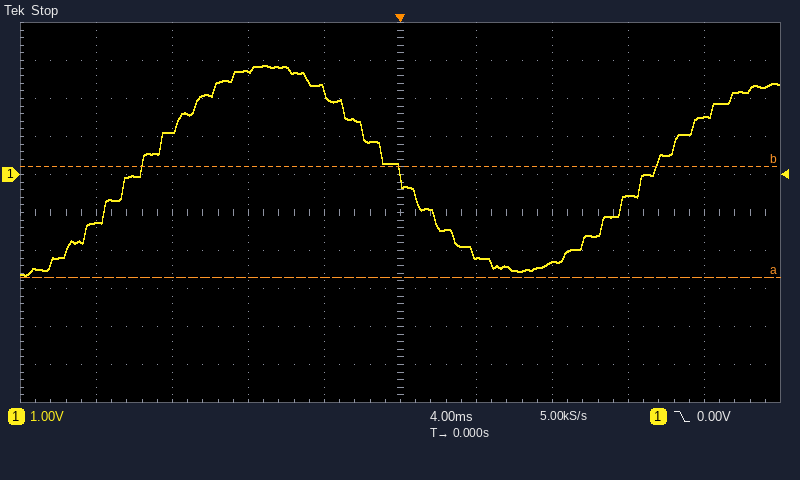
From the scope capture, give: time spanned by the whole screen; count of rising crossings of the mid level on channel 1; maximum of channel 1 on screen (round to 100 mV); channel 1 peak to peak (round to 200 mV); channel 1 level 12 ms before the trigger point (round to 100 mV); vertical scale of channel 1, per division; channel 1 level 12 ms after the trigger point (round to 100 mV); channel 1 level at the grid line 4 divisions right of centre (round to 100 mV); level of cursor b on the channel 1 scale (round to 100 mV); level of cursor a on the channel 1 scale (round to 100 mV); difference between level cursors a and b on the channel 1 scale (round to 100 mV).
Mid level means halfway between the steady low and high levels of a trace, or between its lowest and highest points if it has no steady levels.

40 ms
2
2.9 V
5.6 V
1.2 V
1 V
-600 mV
1.5 V
200 mV
-2.7 V
2.9 V
